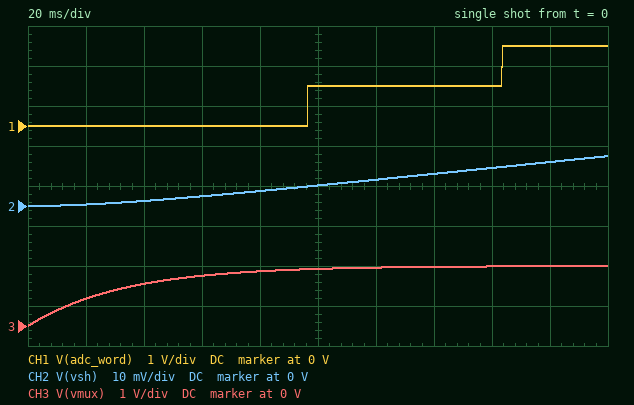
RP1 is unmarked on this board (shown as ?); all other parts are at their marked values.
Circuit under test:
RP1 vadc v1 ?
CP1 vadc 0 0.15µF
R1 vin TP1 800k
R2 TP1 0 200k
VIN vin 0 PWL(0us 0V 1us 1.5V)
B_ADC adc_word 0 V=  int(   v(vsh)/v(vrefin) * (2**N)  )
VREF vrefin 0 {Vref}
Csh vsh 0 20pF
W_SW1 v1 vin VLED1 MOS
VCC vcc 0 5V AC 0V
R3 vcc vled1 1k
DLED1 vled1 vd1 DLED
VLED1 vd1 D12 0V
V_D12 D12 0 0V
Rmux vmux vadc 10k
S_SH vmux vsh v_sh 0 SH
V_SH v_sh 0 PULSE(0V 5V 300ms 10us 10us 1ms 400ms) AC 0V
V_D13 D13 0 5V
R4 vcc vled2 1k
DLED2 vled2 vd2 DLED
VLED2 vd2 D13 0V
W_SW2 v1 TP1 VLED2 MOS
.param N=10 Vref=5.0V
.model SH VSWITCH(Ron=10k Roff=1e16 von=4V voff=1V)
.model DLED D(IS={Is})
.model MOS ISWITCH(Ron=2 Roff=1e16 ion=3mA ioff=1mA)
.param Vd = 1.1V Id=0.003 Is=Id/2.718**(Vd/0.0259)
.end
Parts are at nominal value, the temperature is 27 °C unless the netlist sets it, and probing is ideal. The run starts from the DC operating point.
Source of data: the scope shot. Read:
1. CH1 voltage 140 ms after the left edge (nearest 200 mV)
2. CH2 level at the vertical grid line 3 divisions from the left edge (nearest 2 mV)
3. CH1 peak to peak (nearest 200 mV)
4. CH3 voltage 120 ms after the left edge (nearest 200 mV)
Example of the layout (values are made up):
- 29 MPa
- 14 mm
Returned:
- 1.0 V
- 2 mV
- 2.0 V
- 1.4 V
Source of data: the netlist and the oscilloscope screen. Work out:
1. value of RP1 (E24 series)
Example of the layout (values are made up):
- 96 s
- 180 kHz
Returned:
- 220 kΩ
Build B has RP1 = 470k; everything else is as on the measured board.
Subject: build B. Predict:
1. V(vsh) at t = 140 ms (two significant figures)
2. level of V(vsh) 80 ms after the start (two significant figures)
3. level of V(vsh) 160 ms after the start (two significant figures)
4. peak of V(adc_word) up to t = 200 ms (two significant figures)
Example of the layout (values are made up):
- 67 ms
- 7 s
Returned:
- 5.9 mV
- 2.4 mV
- 7.2 mV
- 2.0 V
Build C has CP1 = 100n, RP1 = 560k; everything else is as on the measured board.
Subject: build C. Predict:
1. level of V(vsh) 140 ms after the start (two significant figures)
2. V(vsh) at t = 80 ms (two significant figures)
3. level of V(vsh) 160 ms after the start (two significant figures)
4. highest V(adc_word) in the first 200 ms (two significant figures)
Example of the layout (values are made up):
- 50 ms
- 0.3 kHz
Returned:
- 6.6 mV
- 2.8 mV
- 8.0 mV
- 2.0 V
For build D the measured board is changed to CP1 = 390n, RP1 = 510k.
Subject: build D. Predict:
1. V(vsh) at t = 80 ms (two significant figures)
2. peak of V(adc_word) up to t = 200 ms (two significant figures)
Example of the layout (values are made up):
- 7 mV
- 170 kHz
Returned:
- 1.1 mV
- 1.0 V
